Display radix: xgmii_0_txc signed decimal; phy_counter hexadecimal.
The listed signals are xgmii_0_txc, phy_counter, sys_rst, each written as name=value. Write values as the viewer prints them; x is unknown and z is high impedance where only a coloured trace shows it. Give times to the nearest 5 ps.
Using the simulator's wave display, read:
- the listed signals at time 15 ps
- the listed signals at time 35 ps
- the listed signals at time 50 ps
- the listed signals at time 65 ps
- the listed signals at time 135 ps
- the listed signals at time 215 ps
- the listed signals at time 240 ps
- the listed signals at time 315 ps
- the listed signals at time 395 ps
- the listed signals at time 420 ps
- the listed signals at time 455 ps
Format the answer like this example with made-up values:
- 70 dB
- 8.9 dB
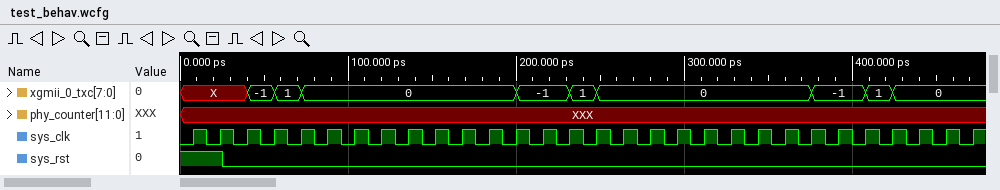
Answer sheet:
- xgmii_0_txc=X, phy_counter=XXX, sys_rst=1
- xgmii_0_txc=X, phy_counter=XXX, sys_rst=0
- xgmii_0_txc=-1, phy_counter=XXX, sys_rst=0
- xgmii_0_txc=1, phy_counter=XXX, sys_rst=0
- xgmii_0_txc=0, phy_counter=XXX, sys_rst=0
- xgmii_0_txc=-1, phy_counter=XXX, sys_rst=0
- xgmii_0_txc=1, phy_counter=XXX, sys_rst=0
- xgmii_0_txc=0, phy_counter=XXX, sys_rst=0
- xgmii_0_txc=-1, phy_counter=XXX, sys_rst=0
- xgmii_0_txc=1, phy_counter=XXX, sys_rst=0
- xgmii_0_txc=0, phy_counter=XXX, sys_rst=0
